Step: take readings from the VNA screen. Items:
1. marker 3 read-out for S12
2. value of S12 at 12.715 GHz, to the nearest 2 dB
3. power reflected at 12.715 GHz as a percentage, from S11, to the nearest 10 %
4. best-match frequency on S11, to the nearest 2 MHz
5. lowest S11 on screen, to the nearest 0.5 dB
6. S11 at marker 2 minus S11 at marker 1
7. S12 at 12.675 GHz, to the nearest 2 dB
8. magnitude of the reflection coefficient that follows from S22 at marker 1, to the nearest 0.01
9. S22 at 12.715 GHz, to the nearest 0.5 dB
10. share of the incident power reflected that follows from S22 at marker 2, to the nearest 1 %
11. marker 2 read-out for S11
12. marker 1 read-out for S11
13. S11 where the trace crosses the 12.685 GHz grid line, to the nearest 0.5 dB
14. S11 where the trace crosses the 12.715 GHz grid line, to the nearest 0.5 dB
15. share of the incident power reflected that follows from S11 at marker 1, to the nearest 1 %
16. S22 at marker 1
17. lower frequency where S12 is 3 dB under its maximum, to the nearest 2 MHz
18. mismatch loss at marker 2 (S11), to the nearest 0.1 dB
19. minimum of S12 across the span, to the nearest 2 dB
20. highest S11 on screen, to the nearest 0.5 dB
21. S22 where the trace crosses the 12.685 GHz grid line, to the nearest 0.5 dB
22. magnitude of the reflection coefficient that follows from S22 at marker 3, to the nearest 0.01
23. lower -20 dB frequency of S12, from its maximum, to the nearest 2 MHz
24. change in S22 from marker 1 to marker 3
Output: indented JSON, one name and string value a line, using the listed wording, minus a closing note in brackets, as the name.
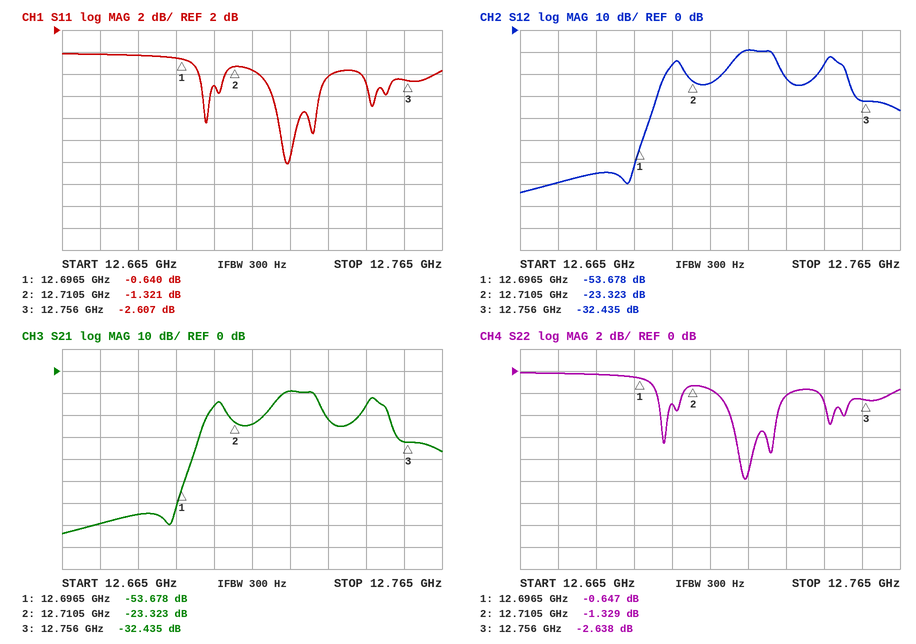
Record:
{
  "marker 3 read-out for S12": "-32.435 dB",
  "value of S12 at 12.715 GHz, to the nearest 2 dB": "-24 dB",
  "power reflected at 12.715 GHz as a percentage, from S11, to the nearest 10 %": "70 %",
  "best-match frequency on S11, to the nearest 2 MHz": "12.724 GHz",
  "lowest S11 on screen, to the nearest 0.5 dB": "-10.0 dB",
  "S11 at marker 2 minus S11 at marker 1": "-0.681 dB",
  "S12 at 12.675 GHz, to the nearest 2 dB": "-70 dB",
  "magnitude of the reflection coefficient that follows from S22 at marker 1, to the nearest 0.01": "0.93",
  "S22 at 12.715 GHz, to the nearest 0.5 dB": "-1.5 dB",
  "share of the incident power reflected that follows from S22 at marker 2, to the nearest 1 %": "74 %",
  "marker 2 read-out for S11": "-1.321 dB",
  "marker 1 read-out for S11": "-0.640 dB",
  "S11 where the trace crosses the 12.685 GHz grid line, to the nearest 0.5 dB": "-0.5 dB",
  "S11 where the trace crosses the 12.715 GHz grid line, to the nearest 0.5 dB": "-1.5 dB",
  "share of the incident power reflected that follows from S11 at marker 1, to the nearest 1 %": "86 %",
  "S22 at marker 1": "-0.647 dB",
  "lower frequency where S12 is 3 dB under its maximum, to the nearest 2 MHz": "12.722 GHz",
  "mismatch loss at marker 2 (S11), to the nearest 0.1 dB": "5.8 dB",
  "minimum of S12 across the span, to the nearest 2 dB": "-74 dB",
  "highest S11 on screen, to the nearest 0.5 dB": "0.0 dB",
  "S22 where the trace crosses the 12.685 GHz grid line, to the nearest 0.5 dB": "-0.5 dB",
  "magnitude of the reflection coefficient that follows from S22 at marker 3, to the nearest 0.01": "0.74",
  "lower -20 dB frequency of S12, from its maximum, to the nearest 2 MHz": "12.702 GHz",
  "change in S22 from marker 1 to marker 3": "-1.991 dB"
}
